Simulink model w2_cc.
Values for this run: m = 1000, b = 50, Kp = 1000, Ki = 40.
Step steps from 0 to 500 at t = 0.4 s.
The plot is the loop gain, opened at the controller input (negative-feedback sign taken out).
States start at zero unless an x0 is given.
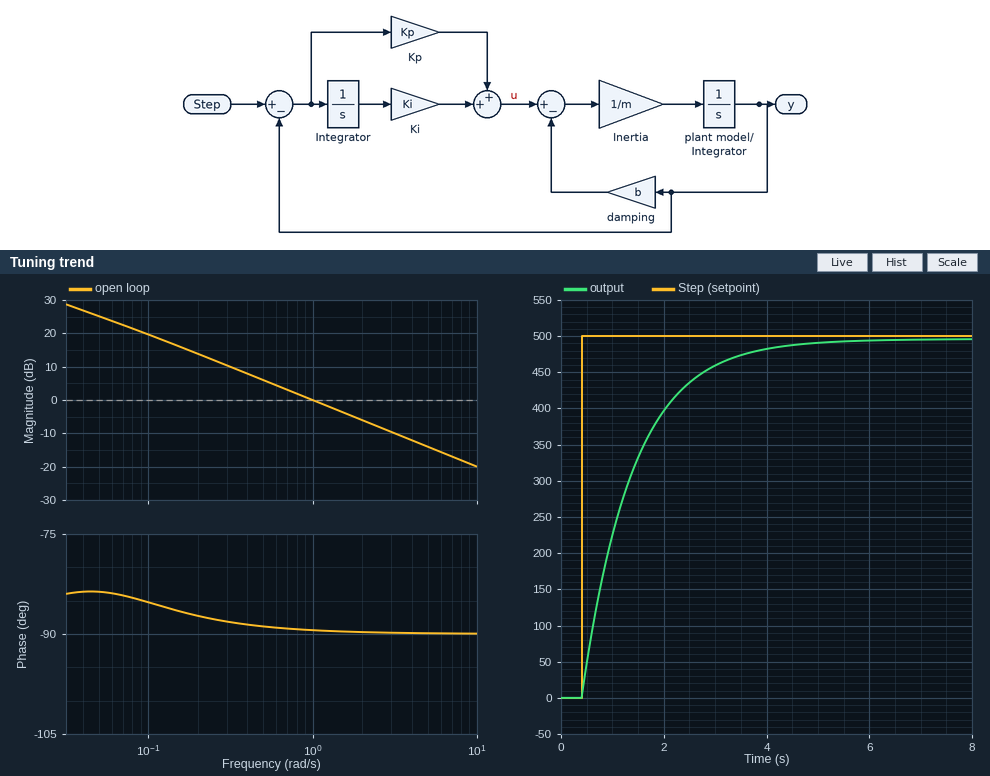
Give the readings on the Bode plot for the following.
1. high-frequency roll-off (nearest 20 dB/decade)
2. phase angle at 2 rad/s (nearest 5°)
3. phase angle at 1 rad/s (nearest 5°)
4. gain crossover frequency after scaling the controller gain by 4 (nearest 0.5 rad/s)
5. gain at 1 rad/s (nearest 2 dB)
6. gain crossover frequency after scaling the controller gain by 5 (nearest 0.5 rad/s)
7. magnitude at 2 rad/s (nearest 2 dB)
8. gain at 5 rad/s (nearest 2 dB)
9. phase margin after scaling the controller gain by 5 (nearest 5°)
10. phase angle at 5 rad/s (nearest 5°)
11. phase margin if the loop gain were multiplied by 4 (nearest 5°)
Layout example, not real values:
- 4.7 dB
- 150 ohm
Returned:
- -20 dB/decade
- -90°
- -90°
- 4.0 rad/s
- 0 dB
- 5.0 rad/s
- -6 dB
- -14 dB
- 90°
- -90°
- 90°
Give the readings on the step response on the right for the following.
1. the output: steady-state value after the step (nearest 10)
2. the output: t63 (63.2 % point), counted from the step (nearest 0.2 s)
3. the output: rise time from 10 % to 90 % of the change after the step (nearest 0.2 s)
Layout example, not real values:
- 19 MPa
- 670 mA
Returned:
- 500
- 1.0 s
- 2.2 s
